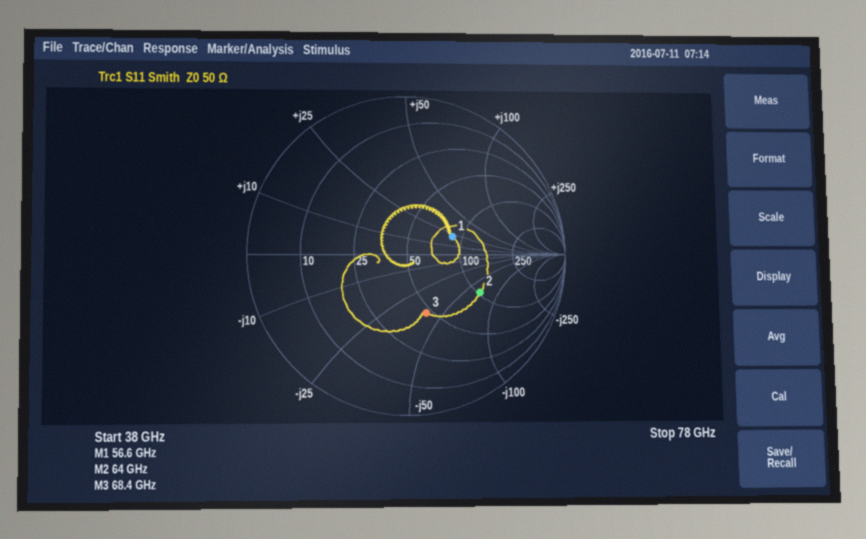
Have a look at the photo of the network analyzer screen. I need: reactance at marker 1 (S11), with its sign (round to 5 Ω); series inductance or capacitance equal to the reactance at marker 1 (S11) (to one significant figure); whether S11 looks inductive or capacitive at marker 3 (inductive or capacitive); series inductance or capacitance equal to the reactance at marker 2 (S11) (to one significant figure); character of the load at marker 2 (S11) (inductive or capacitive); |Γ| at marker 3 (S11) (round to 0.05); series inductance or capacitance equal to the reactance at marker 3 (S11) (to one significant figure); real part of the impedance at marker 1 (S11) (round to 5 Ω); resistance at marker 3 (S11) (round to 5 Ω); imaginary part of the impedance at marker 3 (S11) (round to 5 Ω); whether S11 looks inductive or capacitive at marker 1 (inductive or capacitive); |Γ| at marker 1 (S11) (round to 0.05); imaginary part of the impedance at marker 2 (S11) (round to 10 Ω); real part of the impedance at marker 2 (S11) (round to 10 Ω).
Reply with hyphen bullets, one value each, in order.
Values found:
- +20 Ω
- 60 pH
- capacitive
- 40 fF
- capacitive
- 0.40
- 60 fF
- 85 Ω
- 45 Ω
- -40 Ω
- inductive
- 0.30
- -70 Ω
- 100 Ω
